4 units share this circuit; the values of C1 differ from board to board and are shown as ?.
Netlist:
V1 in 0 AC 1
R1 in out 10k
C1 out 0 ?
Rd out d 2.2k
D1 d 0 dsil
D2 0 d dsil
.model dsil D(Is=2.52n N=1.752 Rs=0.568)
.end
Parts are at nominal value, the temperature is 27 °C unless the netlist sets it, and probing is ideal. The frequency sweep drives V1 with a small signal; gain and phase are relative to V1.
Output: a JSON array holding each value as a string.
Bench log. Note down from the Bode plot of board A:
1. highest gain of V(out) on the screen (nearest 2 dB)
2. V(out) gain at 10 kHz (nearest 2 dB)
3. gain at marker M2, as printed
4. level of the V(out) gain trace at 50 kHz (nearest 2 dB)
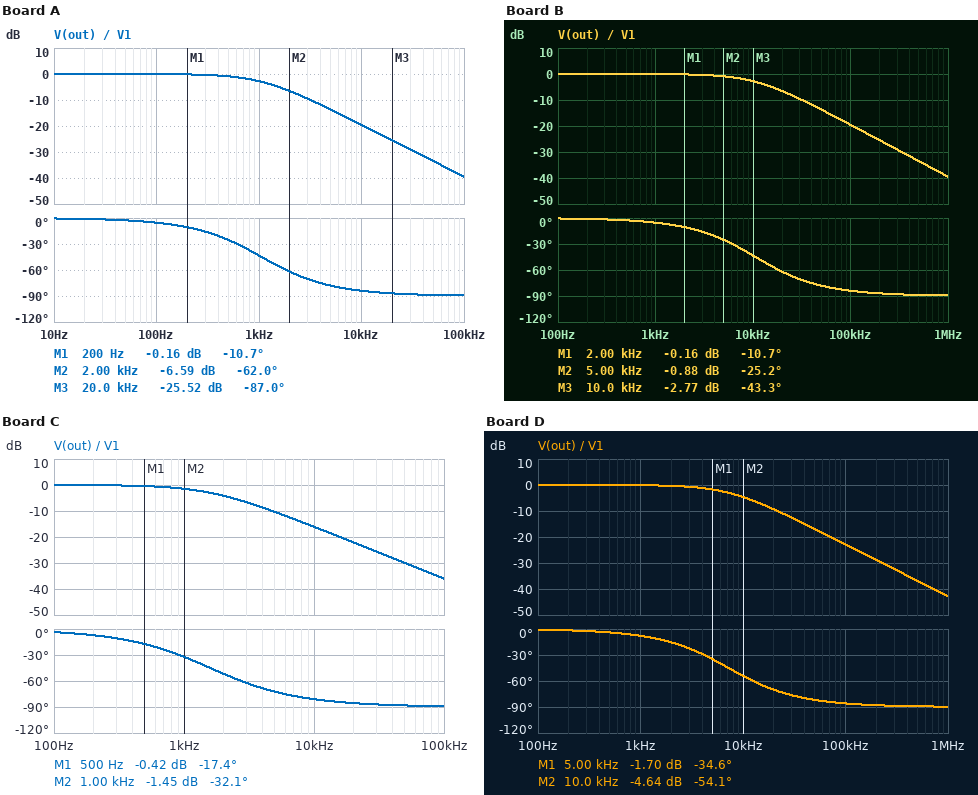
["0 dB", "-20 dB", "-6.59 dB", "-34 dB"]
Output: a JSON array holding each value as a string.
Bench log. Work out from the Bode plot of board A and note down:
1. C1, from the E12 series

["15 nF"]
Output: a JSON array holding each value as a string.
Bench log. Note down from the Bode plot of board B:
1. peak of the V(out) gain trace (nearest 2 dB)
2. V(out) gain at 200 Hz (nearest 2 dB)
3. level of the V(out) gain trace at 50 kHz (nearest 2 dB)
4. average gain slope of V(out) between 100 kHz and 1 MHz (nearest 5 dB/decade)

["0 dB", "0 dB", "-14 dB", "-20 dB/decade"]
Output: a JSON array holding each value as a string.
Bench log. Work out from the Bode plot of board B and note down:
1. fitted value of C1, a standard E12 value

["1.5 nF"]
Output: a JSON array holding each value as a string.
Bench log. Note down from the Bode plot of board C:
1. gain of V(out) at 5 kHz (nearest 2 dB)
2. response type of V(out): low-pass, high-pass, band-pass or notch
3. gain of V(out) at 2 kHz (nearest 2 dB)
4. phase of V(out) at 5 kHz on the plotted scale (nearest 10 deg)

["-10 dB", "low-pass", "-4 dB", "-70 deg"]
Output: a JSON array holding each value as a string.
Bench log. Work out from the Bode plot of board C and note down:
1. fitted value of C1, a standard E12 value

["10 nF"]
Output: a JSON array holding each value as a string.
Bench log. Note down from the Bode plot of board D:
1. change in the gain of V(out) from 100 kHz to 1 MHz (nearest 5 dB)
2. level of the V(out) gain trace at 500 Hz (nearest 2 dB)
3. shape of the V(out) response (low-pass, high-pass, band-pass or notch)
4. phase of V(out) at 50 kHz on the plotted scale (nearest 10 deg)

["-20 dB", "0 dB", "low-pass", "-80 deg"]
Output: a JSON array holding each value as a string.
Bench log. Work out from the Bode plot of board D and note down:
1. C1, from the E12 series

["2.2 nF"]
